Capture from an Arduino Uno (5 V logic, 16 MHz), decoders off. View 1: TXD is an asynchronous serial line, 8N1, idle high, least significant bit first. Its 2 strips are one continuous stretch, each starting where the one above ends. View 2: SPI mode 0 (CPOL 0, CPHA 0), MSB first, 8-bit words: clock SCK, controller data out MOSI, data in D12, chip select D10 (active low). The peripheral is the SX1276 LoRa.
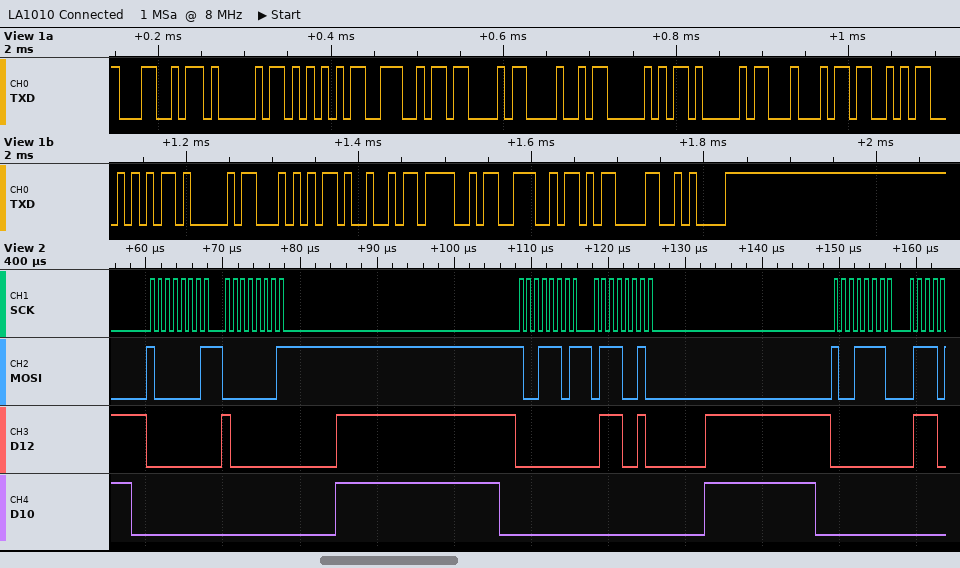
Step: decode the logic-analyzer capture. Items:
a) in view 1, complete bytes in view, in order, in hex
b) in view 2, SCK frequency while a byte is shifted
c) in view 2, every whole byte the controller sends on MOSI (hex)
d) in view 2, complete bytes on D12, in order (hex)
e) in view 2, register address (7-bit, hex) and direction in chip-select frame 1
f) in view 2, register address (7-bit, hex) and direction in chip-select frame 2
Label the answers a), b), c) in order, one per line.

a) 4C 41 55 4E 43 48 50 41 44 53 54 41 54 49 4F 4E 0D 0A
b) 1 MHz
c) 81 01 9D 72 9E
d) 00 80 00 72 00
e) 0x01 write
f) 0x1D write
